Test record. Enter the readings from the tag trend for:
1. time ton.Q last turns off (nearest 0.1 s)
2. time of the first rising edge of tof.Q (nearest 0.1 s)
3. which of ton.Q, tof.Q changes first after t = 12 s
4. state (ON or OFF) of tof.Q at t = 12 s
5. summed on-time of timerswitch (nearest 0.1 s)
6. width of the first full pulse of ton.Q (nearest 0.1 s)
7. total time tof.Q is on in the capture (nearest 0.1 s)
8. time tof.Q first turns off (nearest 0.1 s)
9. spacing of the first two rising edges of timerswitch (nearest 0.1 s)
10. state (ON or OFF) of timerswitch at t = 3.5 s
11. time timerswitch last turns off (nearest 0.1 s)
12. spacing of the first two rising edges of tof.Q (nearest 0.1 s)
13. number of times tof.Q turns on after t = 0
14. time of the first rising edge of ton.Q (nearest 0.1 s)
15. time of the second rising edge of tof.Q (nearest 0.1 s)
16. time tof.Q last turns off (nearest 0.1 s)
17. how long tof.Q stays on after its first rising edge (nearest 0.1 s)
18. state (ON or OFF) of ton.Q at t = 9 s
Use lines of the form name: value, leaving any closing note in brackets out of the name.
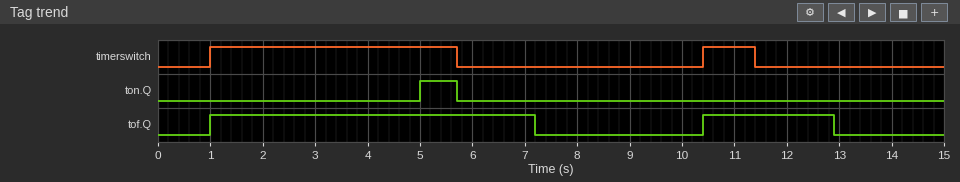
time ton.Q last turns off: 5.7 s
time of the first rising edge of tof.Q: 1.0 s
which of ton.Q, tof.Q changes first after t = 12 s: tof.Q
state (ON or OFF) of tof.Q at t = 12 s: ON
summed on-time of timerswitch: 5.7 s
width of the first full pulse of ton.Q: 0.7 s
total time tof.Q is on in the capture: 8.7 s
time tof.Q first turns off: 7.2 s
spacing of the first two rising edges of timerswitch: 9.4 s
state (ON or OFF) of timerswitch at t = 3.5 s: ON
time timerswitch last turns off: 11.4 s
spacing of the first two rising edges of tof.Q: 9.4 s
number of times tof.Q turns on after t = 0: 2
time of the first rising edge of ton.Q: 5.0 s
time of the second rising edge of tof.Q: 10.4 s
time tof.Q last turns off: 12.9 s
how long tof.Q stays on after its first rising edge: 6.2 s
state (ON or OFF) of ton.Q at t = 9 s: OFF
